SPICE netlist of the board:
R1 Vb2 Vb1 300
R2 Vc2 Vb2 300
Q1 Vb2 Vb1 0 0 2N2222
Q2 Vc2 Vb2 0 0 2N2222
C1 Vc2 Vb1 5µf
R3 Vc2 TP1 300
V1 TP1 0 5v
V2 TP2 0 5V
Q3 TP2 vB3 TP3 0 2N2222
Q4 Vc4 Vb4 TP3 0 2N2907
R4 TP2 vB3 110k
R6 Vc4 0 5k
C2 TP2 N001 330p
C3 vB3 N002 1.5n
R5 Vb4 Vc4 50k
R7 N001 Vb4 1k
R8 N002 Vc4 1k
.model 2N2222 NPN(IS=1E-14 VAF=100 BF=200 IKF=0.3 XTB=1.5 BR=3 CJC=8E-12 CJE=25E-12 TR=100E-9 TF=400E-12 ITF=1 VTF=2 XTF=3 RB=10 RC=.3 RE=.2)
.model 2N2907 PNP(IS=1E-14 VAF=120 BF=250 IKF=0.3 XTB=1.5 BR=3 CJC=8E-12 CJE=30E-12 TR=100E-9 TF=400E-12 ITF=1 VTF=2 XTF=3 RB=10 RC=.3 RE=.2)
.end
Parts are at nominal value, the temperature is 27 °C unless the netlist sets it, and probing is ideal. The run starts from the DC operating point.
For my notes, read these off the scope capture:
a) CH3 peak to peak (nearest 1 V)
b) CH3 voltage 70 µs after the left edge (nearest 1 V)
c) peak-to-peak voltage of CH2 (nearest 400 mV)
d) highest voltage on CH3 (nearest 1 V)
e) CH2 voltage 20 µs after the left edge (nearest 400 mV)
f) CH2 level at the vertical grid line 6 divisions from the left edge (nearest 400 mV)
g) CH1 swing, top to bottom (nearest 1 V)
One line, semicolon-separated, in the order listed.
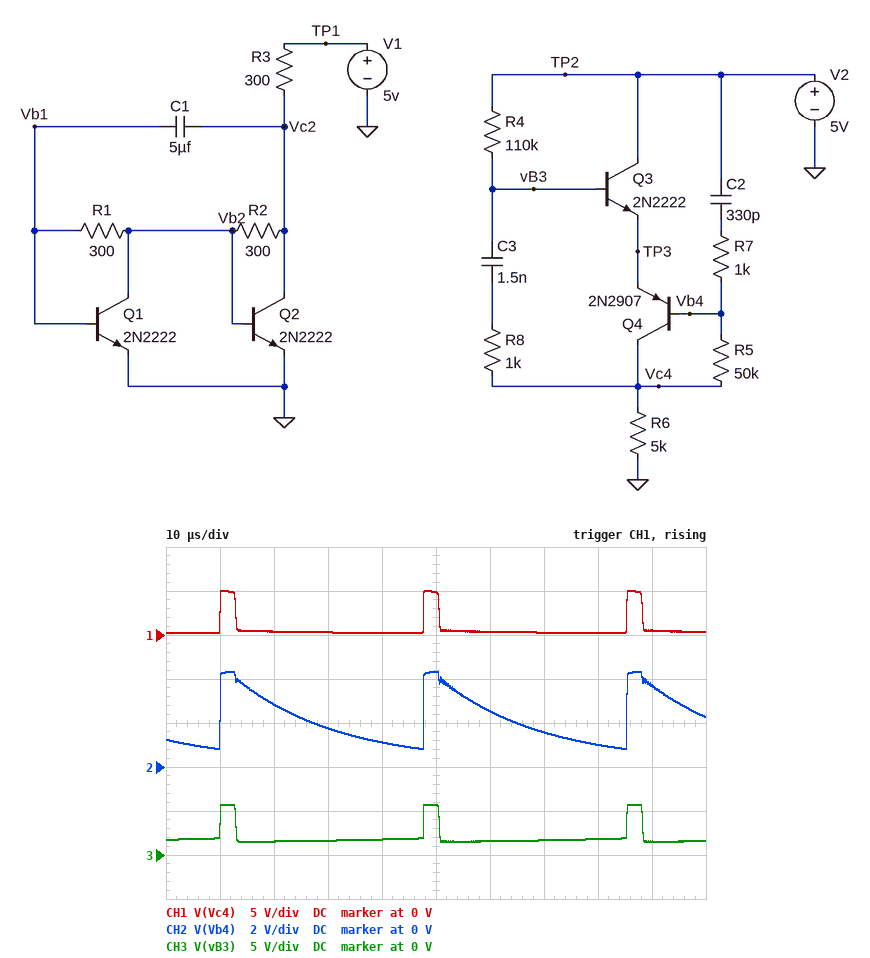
4 V; 2 V; 3.6 V; 6 V; 2.8 V; 2.4 V; 5 V
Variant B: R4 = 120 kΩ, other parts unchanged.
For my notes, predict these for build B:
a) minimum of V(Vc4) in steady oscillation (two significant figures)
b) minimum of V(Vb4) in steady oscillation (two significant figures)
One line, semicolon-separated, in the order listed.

200 mV; 770 mV
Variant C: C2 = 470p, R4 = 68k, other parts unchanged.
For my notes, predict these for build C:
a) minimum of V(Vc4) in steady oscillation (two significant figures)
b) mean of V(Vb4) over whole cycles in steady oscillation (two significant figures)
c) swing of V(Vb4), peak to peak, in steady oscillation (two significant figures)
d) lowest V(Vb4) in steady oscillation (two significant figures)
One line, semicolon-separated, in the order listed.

300 mV; 2.5 V; 3.0 V; 1.3 V
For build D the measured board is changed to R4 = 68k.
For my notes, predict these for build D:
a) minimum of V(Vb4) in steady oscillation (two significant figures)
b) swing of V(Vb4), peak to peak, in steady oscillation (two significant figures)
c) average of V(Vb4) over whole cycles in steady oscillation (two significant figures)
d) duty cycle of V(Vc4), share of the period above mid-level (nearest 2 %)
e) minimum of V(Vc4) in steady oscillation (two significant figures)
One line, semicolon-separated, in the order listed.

1.1 V; 3.2 V; 2.4 V; 10 %; 300 mV
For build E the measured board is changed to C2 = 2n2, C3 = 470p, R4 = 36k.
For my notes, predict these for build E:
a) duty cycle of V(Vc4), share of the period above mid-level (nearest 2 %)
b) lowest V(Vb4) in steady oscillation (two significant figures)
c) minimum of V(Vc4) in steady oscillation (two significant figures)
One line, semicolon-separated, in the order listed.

10 %; 3.1 V; 400 mV
